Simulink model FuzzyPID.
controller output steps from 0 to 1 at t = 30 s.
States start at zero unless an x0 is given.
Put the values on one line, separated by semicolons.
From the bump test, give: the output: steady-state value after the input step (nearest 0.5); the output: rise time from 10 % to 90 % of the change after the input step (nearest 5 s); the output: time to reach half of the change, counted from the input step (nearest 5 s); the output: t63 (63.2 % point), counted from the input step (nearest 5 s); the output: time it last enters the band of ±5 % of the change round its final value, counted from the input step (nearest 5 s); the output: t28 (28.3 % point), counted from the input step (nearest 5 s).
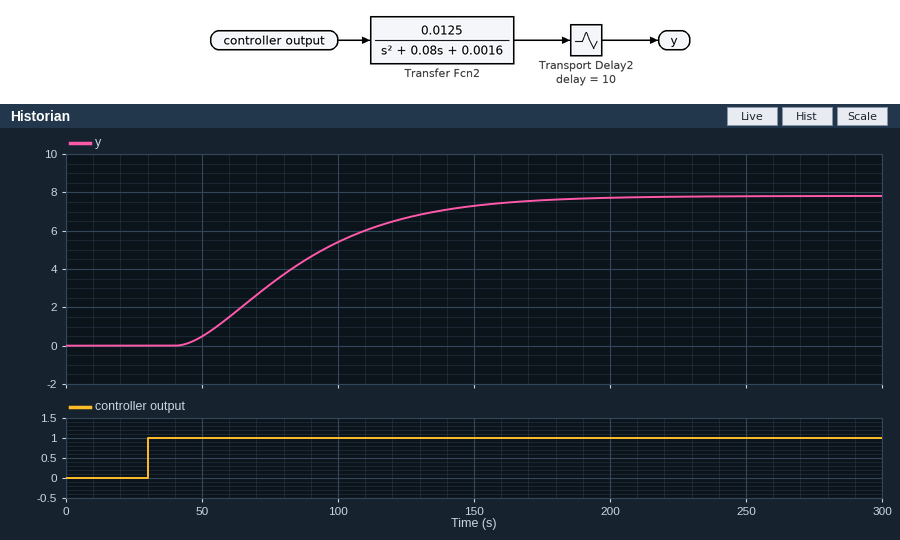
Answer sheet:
8.0; 85 s; 50 s; 65 s; 130 s; 35 s
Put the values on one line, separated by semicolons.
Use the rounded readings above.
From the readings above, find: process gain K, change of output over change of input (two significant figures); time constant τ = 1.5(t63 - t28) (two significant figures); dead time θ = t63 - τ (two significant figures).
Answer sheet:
8.0; 45 s; 20 s
